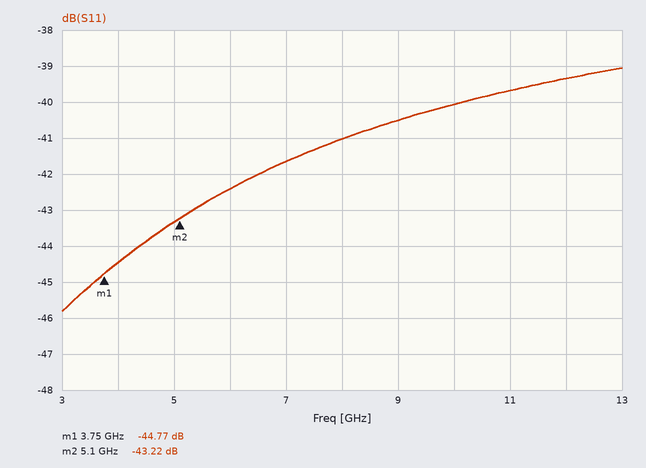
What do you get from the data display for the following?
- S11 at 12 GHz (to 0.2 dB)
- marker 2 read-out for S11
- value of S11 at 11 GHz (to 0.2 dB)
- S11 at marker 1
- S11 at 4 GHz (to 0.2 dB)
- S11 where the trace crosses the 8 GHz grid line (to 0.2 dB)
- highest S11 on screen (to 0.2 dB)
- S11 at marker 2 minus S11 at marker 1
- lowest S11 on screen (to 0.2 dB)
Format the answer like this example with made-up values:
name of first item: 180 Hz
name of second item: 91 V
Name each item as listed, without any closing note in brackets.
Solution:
S11 at 12 GHz: -39.4 dB
marker 2 read-out for S11: -43.22 dB
value of S11 at 11 GHz: -39.6 dB
S11 at marker 1: -44.77 dB
S11 at 4 GHz: -44.4 dB
S11 where the trace crosses the 8 GHz grid line: -41.0 dB
highest S11 on screen: -39.0 dB
S11 at marker 2 minus S11 at marker 1: 1.55 dB
lowest S11 on screen: -45.8 dB
